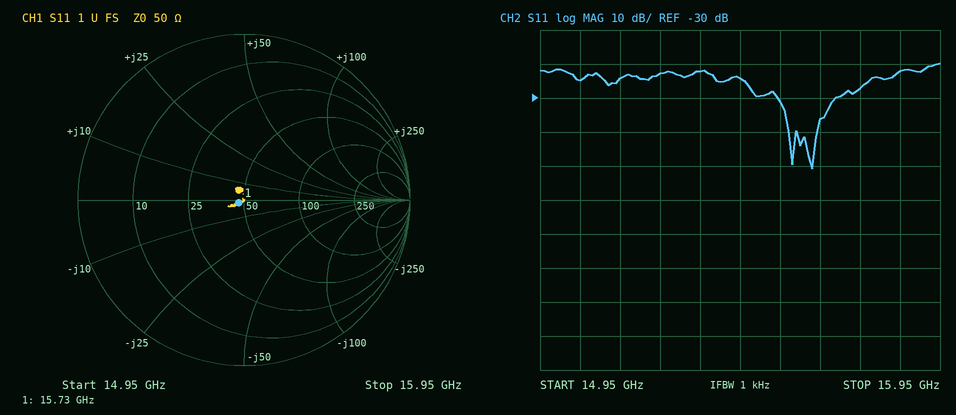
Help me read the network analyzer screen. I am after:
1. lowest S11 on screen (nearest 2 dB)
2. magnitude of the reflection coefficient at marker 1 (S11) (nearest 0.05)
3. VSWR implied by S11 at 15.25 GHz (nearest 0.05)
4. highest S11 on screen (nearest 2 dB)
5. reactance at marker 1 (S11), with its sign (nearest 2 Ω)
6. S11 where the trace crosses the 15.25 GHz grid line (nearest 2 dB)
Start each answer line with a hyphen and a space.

- -50 dB
- 0.05
- 1.15
- -20 dB
- -2 Ω
- -22 dB
